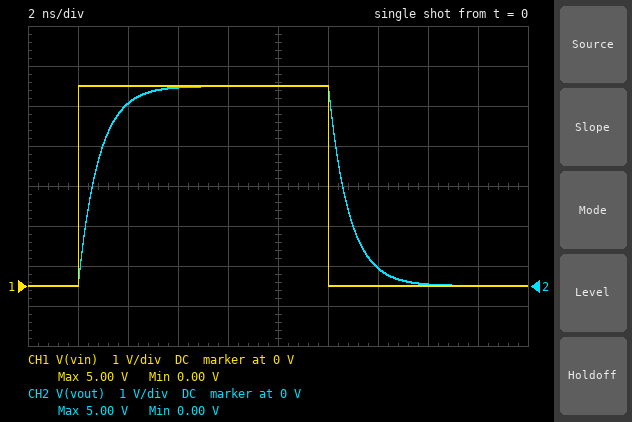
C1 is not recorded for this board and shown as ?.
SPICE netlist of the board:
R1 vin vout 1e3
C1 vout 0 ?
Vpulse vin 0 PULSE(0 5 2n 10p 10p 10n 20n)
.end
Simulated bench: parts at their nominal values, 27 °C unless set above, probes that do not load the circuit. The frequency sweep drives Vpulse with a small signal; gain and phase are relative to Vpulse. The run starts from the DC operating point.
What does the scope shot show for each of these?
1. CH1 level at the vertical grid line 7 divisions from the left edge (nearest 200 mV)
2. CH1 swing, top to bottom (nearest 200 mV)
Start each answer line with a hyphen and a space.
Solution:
- 0 V
- 5.0 V
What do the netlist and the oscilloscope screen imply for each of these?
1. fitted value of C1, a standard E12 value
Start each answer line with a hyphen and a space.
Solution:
- 820 fF
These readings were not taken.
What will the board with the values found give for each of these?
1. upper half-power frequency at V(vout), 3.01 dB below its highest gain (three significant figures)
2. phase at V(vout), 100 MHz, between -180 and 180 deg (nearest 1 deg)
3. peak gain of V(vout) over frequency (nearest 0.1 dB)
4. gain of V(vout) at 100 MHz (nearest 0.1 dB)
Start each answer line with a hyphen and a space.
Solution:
- 194 MHz
- -27 deg
- 0 dB
- -1.0 dB
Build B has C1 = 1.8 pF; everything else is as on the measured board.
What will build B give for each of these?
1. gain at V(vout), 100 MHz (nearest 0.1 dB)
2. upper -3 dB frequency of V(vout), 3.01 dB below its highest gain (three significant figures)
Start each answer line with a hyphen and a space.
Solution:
- -3.6 dB
- 88.4 MHz
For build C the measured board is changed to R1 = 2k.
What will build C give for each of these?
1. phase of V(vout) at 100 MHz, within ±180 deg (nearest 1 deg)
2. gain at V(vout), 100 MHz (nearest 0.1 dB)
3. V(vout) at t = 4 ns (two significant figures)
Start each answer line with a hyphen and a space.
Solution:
- -46 deg
- -3.1 dB
- 3.5 V
